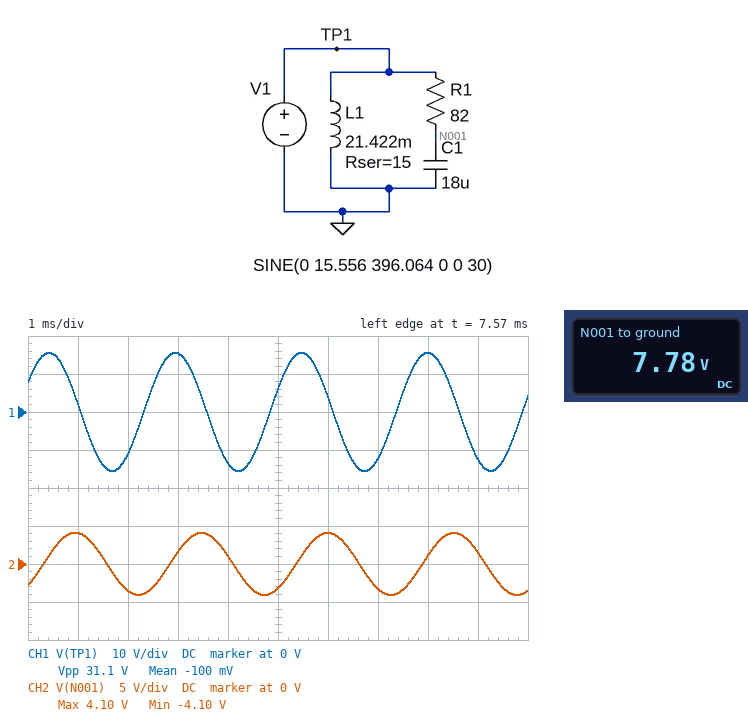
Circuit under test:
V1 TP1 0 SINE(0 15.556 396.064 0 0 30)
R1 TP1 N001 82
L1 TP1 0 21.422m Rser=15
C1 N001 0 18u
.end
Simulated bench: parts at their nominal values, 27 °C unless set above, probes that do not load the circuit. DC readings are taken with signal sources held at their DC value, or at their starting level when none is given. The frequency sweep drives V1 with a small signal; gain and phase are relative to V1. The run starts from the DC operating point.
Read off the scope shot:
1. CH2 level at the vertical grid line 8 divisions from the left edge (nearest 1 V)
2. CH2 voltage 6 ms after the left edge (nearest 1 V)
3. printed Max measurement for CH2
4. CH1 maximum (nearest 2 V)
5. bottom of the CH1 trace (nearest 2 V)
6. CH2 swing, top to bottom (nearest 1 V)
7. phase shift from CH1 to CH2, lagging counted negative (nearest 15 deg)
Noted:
1 V
4 V
4.10 V
16 V
-16 V
8 V
-75 deg
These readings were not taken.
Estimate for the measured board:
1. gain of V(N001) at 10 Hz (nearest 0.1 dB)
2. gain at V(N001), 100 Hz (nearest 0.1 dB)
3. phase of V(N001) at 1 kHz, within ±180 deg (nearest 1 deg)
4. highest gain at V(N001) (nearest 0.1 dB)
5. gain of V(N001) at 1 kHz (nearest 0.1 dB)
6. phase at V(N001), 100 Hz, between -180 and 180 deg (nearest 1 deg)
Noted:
0 dB
-2.7 dB
-84 deg
0 dB
-19.4 dB
-43 deg
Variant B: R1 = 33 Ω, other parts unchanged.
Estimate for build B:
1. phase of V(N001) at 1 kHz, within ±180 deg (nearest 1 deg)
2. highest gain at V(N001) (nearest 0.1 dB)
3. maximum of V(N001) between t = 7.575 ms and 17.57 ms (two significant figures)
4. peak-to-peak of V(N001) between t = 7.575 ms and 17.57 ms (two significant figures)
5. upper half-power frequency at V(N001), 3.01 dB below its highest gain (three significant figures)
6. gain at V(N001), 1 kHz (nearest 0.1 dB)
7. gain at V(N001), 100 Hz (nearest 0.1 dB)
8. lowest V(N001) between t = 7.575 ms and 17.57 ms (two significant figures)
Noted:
-75 deg
0 dB
8.7 V
17 V
268 Hz
-11.7 dB
-0.6 dB
-8.7 V
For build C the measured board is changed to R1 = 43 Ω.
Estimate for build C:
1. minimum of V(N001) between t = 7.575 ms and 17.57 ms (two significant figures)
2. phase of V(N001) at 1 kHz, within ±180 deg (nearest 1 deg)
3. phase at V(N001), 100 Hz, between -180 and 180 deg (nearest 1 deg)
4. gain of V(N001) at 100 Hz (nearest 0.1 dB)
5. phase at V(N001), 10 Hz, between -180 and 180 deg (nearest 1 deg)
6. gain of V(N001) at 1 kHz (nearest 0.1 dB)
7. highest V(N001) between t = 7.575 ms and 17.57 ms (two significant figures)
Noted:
-7.2 V
-78 deg
-26 deg
-0.9 dB
-3 deg
-13.9 dB
7.2 V
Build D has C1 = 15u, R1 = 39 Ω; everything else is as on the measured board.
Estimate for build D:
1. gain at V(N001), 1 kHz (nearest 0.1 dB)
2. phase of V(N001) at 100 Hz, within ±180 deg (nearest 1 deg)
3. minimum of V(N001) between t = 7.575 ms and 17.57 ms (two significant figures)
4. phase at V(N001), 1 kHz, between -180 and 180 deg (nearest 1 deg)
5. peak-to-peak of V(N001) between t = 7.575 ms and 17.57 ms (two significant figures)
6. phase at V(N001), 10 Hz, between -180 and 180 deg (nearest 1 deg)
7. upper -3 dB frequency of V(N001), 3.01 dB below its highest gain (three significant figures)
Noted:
-11.6 dB
-20 deg
-8.8 V
-75 deg
18 V
-2 deg
272 Hz
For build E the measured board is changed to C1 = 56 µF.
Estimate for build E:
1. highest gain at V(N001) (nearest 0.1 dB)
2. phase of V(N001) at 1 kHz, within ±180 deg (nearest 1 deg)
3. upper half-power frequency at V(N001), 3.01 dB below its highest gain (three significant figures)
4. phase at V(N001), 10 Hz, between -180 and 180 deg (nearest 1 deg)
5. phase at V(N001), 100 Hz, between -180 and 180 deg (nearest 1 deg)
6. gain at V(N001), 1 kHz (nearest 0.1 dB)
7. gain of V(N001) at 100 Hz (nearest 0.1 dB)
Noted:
0 dB
-88 deg
34.7 Hz
-16 deg
-71 deg
-29.2 dB
-9.7 dB
